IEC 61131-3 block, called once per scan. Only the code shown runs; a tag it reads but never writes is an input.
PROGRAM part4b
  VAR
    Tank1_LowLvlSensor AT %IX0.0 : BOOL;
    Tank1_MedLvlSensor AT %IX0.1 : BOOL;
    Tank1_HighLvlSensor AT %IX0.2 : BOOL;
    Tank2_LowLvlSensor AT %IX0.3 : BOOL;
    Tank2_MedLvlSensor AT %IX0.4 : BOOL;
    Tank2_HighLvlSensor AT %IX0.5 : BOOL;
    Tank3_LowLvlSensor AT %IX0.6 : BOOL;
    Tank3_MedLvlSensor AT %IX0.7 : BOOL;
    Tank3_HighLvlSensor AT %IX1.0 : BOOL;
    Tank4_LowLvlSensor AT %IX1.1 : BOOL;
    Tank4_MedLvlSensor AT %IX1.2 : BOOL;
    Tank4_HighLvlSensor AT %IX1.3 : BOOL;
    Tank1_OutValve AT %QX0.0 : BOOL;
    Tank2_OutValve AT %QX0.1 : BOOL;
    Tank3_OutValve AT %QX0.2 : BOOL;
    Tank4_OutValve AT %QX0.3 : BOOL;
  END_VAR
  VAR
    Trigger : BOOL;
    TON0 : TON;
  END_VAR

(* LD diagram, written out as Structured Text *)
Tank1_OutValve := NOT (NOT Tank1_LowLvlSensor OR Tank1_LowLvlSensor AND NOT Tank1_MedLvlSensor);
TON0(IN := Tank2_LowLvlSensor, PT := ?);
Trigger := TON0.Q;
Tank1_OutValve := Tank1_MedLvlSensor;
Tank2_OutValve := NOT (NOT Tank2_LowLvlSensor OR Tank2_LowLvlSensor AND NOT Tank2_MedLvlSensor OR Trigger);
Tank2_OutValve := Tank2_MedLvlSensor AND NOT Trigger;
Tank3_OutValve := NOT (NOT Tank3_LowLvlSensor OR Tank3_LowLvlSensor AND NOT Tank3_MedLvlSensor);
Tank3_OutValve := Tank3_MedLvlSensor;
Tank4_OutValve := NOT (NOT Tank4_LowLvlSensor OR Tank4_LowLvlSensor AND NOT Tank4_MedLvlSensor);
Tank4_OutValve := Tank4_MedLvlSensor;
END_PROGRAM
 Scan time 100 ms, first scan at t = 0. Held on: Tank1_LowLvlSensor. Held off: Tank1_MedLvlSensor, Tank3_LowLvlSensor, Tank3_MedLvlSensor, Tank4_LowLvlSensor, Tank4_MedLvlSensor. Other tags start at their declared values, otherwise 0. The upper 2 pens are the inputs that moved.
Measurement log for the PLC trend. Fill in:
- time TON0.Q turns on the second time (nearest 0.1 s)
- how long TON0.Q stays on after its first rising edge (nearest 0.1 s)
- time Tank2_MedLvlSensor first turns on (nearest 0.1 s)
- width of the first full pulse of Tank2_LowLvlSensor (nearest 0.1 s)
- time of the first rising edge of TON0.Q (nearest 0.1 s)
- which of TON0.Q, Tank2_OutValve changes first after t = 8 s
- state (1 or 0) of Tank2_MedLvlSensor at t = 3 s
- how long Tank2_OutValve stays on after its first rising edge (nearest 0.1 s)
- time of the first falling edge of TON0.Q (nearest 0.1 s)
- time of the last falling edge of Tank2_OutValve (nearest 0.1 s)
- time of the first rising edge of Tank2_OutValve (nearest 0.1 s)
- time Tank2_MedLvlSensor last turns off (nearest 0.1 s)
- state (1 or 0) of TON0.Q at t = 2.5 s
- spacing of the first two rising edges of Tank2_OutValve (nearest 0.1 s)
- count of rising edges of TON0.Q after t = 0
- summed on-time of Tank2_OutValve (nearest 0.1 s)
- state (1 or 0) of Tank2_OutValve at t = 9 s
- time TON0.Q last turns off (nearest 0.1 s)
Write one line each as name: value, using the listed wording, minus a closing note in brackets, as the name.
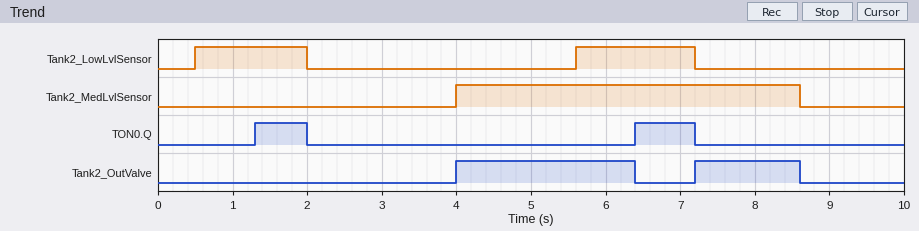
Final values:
time TON0.Q turns on the second time: 6.4 s
how long TON0.Q stays on after its first rising edge: 0.7 s
time Tank2_MedLvlSensor first turns on: 4.0 s
width of the first full pulse of Tank2_LowLvlSensor: 1.5 s
time of the first rising edge of TON0.Q: 1.3 s
which of TON0.Q, Tank2_OutValve changes first after t = 8 s: Tank2_OutValve
state (1 or 0) of Tank2_MedLvlSensor at t = 3 s: 0
how long Tank2_OutValve stays on after its first rising edge: 2.4 s
time of the first falling edge of TON0.Q: 2.0 s
time of the last falling edge of Tank2_OutValve: 8.6 s
time of the first rising edge of Tank2_OutValve: 4.0 s
time Tank2_MedLvlSensor last turns off: 8.6 s
state (1 or 0) of TON0.Q at t = 2.5 s: 0
spacing of the first two rising edges of Tank2_OutValve: 3.2 s
count of rising edges of TON0.Q after t = 0: 2
summed on-time of Tank2_OutValve: 3.8 s
state (1 or 0) of Tank2_OutValve at t = 9 s: 0
time TON0.Q last turns off: 7.2 s
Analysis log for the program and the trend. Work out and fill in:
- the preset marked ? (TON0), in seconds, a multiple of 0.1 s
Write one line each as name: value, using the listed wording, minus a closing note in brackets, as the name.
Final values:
the preset marked ? (TON0), in seconds, a multiple of 0.1 s: 0.8 s
